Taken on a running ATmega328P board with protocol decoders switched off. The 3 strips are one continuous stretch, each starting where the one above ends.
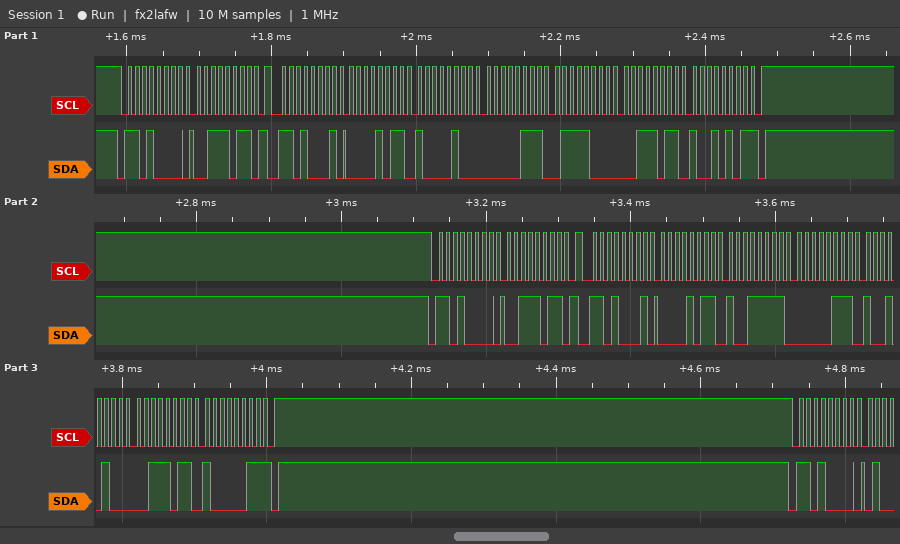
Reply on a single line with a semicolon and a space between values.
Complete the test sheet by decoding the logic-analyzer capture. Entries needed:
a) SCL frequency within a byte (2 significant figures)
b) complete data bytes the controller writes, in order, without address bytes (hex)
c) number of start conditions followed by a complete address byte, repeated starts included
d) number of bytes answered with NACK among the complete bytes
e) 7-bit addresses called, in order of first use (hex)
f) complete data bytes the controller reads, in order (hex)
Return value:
100 kHz; 3B 3B; 5; 2; 0x68; 0B 84 07 78 3B 95 0B 9F 07 94 3B 83
